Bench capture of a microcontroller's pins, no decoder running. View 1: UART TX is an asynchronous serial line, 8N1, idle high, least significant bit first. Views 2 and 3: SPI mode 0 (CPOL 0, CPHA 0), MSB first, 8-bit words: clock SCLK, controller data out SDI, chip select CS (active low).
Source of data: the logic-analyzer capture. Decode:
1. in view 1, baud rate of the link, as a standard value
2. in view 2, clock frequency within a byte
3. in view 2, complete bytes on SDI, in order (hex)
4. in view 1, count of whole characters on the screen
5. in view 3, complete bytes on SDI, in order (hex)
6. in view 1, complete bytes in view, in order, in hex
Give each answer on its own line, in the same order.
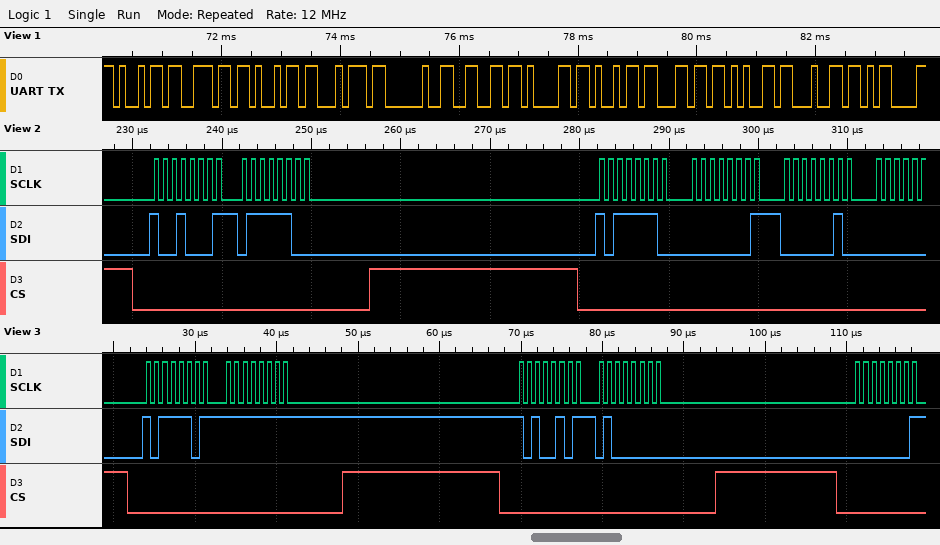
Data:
9600 baud
1 MHz
91 7C BE 01 02
12
BD FF A5 40 01
69 6E 69 74 20 66 61 69 6C 65 64 0D
